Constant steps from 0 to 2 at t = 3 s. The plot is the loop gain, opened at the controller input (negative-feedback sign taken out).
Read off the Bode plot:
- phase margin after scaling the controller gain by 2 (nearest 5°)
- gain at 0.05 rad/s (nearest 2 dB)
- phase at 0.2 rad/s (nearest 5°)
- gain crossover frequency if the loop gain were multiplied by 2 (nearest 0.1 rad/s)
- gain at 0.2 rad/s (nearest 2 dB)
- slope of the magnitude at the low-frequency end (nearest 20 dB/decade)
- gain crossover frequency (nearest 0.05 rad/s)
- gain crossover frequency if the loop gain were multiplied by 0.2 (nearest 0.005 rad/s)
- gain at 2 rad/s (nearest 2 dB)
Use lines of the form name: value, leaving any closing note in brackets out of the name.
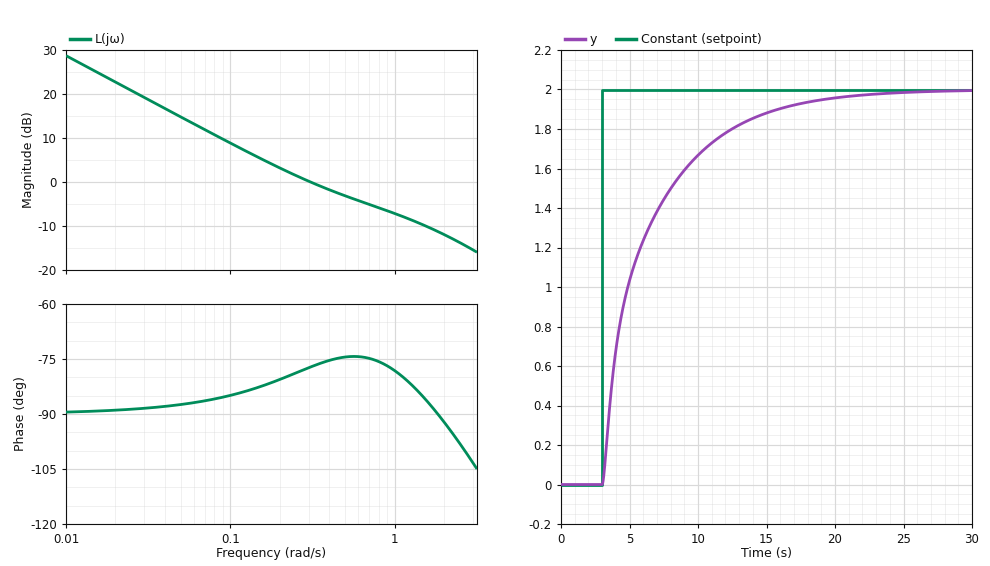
phase margin after scaling the controller gain by 2: 105°
gain at 0.05 rad/s: 14 dB
phase at 0.2 rad/s: -80°
gain crossover frequency if the loop gain were multiplied by 2: 0.8 rad/s
gain at 0.2 rad/s: 4 dB
slope of the magnitude at the low-frequency end: -20 dB/decade
gain crossover frequency: 0.30 rad/s
gain crossover frequency if the loop gain were multiplied by 0.2: 0.055 rad/s
gain at 2 rad/s: -12 dB
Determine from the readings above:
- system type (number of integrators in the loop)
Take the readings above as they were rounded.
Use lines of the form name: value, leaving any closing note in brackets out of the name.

system type: 1
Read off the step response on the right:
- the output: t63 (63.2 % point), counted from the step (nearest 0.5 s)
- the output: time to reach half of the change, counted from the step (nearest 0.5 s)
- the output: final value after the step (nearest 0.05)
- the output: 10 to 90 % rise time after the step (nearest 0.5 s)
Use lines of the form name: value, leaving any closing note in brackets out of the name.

the output: t63 (63.2 % point), counted from the step: 3.0 s
the output: time to reach half of the change, counted from the step: 2.0 s
the output: final value after the step: 2.00
the output: 10 to 90 % rise time after the step: 9.0 s
